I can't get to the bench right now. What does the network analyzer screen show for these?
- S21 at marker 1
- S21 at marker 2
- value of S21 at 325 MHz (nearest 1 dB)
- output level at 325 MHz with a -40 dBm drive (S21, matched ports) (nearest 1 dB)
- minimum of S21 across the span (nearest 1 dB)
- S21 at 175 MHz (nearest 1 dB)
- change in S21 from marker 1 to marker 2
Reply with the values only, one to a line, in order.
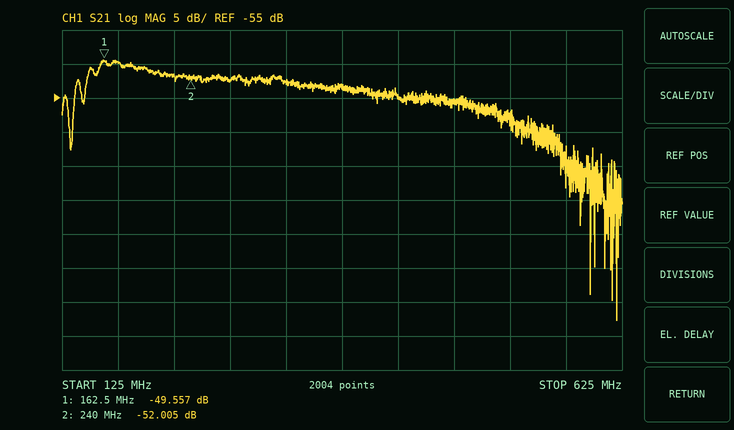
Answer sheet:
-49.557 dB
-52.005 dB
-53 dB
-93 dBm
-88 dB
-50 dB
-2.448 dB
